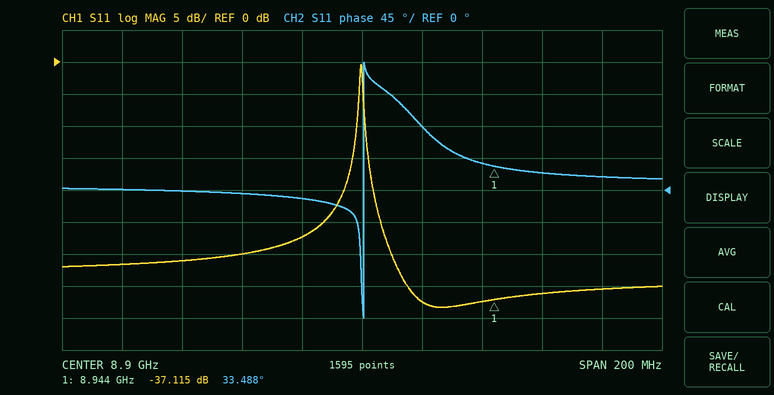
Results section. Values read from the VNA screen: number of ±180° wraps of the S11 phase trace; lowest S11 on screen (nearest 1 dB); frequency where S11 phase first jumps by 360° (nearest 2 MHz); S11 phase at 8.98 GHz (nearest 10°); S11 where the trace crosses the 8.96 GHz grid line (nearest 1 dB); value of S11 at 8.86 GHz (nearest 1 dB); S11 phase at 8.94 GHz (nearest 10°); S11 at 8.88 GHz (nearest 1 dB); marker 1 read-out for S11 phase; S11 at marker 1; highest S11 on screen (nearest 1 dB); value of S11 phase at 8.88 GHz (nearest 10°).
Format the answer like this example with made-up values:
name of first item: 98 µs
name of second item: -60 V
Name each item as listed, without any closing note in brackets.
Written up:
number of ±180° wraps of the S11 phase trace: 1
lowest S11 on screen: -38 dB
frequency where S11 phase first jumps by 360°: 8.900 GHz
S11 phase at 8.98 GHz: 20°
S11 where the trace crosses the 8.96 GHz grid line: -36 dB
value of S11 at 8.86 GHz: -30 dB
S11 phase at 8.94 GHz: 40°
S11 at 8.88 GHz: -27 dB
marker 1 read-out for S11 phase: 33.488°
S11 at marker 1: -37.115 dB
highest S11 on screen: 0 dB
value of S11 phase at 8.88 GHz: -10°
